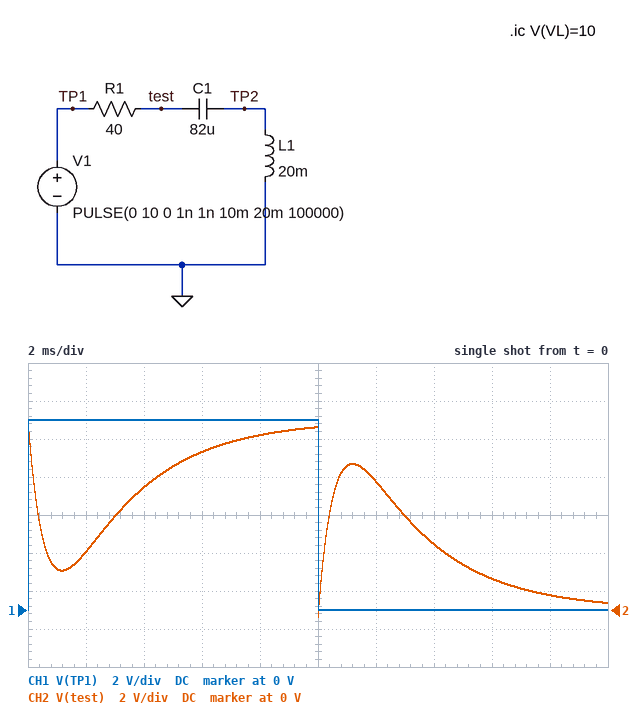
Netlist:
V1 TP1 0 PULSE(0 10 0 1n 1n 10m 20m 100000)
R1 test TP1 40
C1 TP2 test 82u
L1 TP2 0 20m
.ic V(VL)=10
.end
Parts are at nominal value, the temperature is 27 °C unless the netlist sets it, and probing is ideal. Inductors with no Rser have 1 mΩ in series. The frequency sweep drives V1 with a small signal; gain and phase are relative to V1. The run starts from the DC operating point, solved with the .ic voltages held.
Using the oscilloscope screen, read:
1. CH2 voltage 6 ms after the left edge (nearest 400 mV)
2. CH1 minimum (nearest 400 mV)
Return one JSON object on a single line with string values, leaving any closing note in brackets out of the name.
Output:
{"CH2 voltage 6 ms after the left edge": "8.4 V", "CH1 minimum": "0 V"}
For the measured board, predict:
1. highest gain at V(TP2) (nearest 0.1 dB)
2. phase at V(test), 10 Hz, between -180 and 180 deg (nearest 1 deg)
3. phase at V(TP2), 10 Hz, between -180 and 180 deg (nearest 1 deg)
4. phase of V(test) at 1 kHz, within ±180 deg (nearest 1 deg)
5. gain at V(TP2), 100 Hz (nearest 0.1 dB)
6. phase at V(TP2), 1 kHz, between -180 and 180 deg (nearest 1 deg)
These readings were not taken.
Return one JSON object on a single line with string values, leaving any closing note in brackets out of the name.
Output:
{"highest gain at V(TP2)": "0 dB", "phase at V(test), 10 Hz, between -180 and 180 deg": "-12 deg", "phase at V(TP2), 10 Hz, between -180 and 180 deg": "168 deg", "phase of V(test) at 1 kHz, within ±180 deg": "18 deg", "gain at V(TP2), 100 Hz": "-10.2 dB", "phase at V(TP2), 1 kHz, between -180 and 180 deg": "18 deg"}
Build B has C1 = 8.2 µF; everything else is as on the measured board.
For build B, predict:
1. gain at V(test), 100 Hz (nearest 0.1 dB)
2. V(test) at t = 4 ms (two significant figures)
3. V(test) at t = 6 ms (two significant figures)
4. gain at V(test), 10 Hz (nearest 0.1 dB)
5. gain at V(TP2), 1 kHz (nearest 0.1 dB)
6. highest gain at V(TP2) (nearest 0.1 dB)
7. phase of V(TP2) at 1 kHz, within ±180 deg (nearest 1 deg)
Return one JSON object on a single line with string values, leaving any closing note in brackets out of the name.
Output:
{"gain at V(test), 100 Hz": "-0.2 dB", "V(test) at t = 4 ms": "9.9 V", "V(test) at t = 6 ms": "10 V", "gain at V(test), 10 Hz": "0 dB", "gain at V(TP2), 1 kHz": "0.9 dB", "highest gain at V(TP2)": "2.6 dB", "phase of V(TP2) at 1 kHz, within ±180 deg": "21 deg"}
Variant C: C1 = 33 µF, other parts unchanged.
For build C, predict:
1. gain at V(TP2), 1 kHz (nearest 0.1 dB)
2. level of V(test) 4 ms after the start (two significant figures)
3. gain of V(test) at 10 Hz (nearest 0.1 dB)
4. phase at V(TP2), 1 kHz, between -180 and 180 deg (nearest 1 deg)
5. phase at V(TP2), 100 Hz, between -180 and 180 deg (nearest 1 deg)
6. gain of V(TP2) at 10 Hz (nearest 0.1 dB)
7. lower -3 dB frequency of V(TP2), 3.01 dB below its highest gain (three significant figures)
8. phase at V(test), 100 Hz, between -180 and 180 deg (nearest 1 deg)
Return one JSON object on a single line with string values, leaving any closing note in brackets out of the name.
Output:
{"gain at V(TP2), 1 kHz": "-0.1 dB", "level of V(test) 4 ms after the start": "9.9 V", "gain of V(test) at 10 Hz": "0 dB", "phase at V(TP2), 1 kHz, between -180 and 180 deg": "18 deg", "phase at V(TP2), 100 Hz, between -180 and 180 deg": "132 deg", "gain of V(TP2) at 10 Hz": "-51.7 dB", "lower -3 dB frequency of V(TP2), 3.01 dB below its highest gain": "229 Hz", "phase at V(test), 100 Hz, between -180 and 180 deg": "-48 deg"}
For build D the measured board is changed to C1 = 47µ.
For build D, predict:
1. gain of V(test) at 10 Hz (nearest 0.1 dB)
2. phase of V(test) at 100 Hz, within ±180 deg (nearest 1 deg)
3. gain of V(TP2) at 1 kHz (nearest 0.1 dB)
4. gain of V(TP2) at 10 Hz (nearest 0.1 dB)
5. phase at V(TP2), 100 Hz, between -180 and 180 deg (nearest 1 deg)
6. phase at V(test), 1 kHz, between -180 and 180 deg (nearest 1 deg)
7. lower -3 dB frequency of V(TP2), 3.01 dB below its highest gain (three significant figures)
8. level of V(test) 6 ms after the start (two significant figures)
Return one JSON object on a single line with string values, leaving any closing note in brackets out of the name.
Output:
{"gain of V(test) at 10 Hz": "-0.1 dB", "phase of V(test) at 100 Hz, within ±180 deg": "-62 deg", "gain of V(TP2) at 1 kHz": "-0.2 dB", "gain of V(TP2) at 10 Hz": "-48.6 dB", "phase at V(TP2), 100 Hz, between -180 and 180 deg": "118 deg", "phase at V(test), 1 kHz, between -180 and 180 deg": "18 deg", "lower -3 dB frequency of V(TP2), 3.01 dB below its highest gain": "244 Hz", "level of V(test) 6 ms after the start": "9.8 V"}
